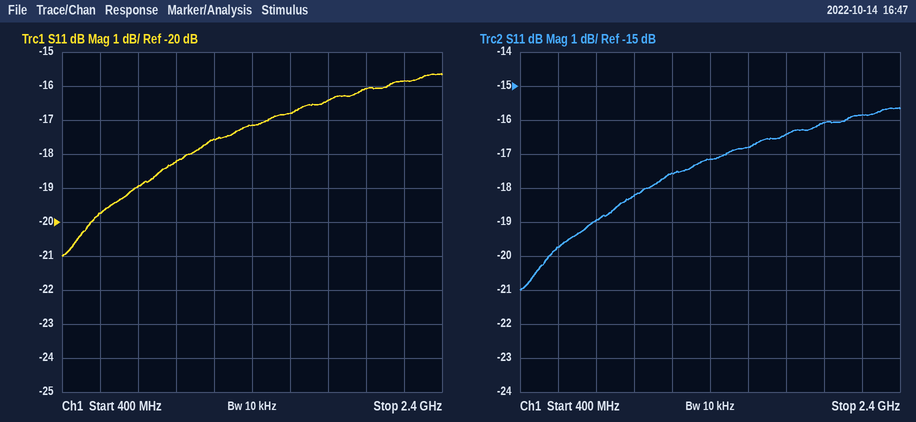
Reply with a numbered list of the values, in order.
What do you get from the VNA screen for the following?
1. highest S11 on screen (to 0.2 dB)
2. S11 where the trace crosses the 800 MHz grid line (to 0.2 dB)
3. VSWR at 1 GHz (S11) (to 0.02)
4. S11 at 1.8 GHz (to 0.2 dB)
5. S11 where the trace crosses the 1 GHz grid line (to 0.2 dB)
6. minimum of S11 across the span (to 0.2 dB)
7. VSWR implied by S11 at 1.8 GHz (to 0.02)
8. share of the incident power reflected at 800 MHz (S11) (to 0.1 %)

1. -15.6 dB
2. -19.0 dB
3. 1.28
4. -16.4 dB
5. -18.2 dB
6. -21.0 dB
7. 1.36
8. 1.3 %
